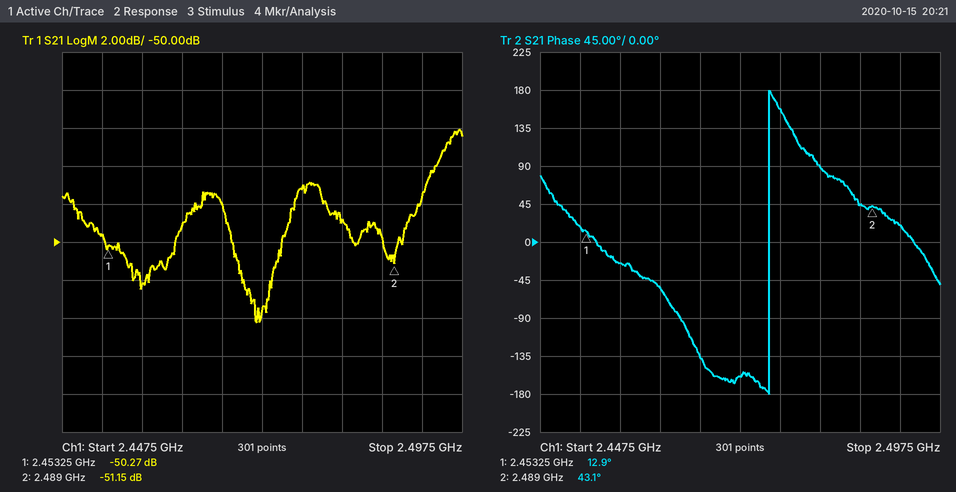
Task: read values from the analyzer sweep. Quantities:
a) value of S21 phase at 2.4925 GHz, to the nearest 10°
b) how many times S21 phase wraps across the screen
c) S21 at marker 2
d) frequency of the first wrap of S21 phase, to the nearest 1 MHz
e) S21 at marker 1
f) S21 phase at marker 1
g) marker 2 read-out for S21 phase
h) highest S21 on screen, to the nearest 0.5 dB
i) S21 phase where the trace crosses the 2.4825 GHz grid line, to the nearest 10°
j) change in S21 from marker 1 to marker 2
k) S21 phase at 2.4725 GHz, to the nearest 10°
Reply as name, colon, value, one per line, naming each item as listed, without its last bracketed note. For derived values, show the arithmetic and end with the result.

value of S21 phase at 2.4925 GHz, to the nearest 10°: 20°
how many times S21 phase wraps across the screen: 1
S21 at marker 2: -51.15 dB
frequency of the first wrap of S21 phase, to the nearest 1 MHz: 2.476 GHz
S21 at marker 1: -50.27 dB
S21 phase at marker 1: 12.9°
marker 2 read-out for S21 phase: 43.1°
highest S21 on screen, to the nearest 0.5 dB: -44.0 dB
S21 phase where the trace crosses the 2.4825 GHz grid line, to the nearest 10°: 90°
change in S21 from marker 1 to marker 2: -51.15 − (-50.27) = -0.88 dB
S21 phase at 2.4725 GHz, to the nearest 10°: -160°
